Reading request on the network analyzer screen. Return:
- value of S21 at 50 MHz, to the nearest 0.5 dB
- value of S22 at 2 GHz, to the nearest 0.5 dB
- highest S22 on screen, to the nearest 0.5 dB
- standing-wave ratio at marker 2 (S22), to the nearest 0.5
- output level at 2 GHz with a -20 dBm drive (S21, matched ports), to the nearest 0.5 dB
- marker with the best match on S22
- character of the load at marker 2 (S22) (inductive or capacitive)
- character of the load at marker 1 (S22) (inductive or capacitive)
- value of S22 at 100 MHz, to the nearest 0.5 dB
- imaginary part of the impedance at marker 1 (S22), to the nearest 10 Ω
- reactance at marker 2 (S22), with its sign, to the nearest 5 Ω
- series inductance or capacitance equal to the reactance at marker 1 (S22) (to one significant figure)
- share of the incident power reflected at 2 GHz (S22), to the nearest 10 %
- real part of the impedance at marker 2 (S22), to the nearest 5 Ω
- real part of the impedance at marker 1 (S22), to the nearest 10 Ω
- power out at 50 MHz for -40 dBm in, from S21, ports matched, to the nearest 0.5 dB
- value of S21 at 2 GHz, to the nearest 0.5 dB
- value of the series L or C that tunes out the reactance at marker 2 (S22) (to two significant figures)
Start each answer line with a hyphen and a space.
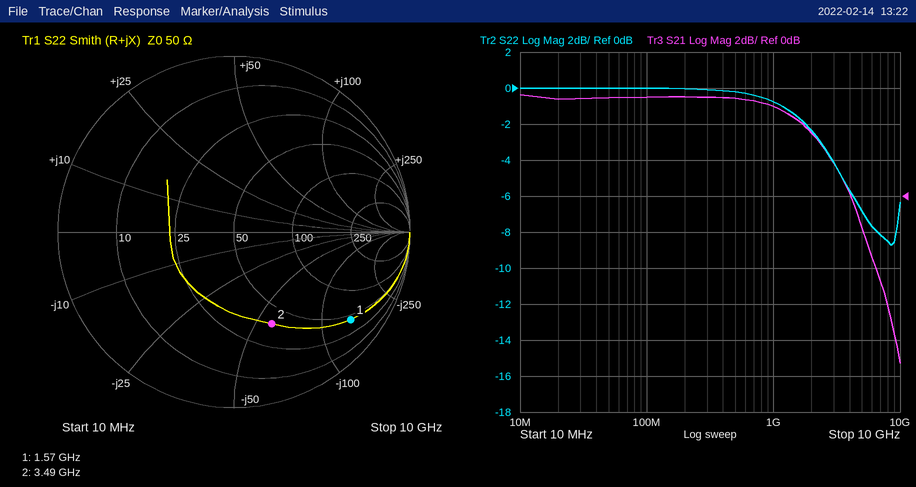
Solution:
- 5.5 dB
- -2.5 dB
- 0.0 dB
- 3.5
- -16.5 dBm
- marker 2
- capacitive
- capacitive
- 0.0 dB
- -140 Ω
- -60 Ω
- 700 fF
- 60 %
- 40 Ω
- 40 Ω
- -34.5 dBm
- 3.5 dB
- 2.7 nH
